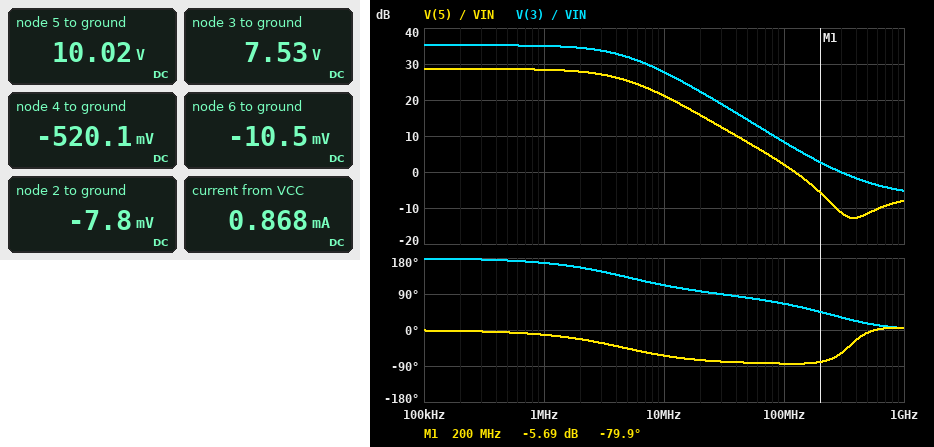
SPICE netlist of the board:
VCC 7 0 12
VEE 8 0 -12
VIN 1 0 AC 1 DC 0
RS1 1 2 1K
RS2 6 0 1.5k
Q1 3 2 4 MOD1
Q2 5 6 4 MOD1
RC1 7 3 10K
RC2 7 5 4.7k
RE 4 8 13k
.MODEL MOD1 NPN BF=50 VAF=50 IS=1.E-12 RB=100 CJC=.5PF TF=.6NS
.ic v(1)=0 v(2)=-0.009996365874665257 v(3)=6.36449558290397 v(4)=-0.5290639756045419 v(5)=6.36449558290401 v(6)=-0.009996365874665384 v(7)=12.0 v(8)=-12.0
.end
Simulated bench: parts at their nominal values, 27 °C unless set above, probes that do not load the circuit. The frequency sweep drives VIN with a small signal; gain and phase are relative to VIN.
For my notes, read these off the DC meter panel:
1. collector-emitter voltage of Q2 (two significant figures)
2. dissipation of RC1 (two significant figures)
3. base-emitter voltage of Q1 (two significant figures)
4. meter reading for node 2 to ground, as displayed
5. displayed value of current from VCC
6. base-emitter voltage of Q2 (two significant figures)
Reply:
11 V
2.0 mW
510 mV
-7.8 mV
0.868 mA
510 mV
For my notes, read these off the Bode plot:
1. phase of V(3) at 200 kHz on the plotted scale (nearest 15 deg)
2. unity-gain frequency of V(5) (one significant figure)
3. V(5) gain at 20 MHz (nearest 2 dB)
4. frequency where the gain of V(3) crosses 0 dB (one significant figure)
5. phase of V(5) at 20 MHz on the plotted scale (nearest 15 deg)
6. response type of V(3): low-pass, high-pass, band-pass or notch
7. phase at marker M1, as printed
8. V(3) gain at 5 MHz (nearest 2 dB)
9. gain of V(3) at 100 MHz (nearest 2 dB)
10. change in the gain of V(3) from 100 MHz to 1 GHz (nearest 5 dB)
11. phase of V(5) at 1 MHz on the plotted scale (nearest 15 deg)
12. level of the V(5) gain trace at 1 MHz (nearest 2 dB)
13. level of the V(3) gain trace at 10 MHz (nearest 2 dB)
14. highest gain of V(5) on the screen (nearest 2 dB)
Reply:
180 deg
100 MHz
16 dB
300 MHz
-75 deg
low-pass
-79.9 deg
32 dB
8 dB
-15 dB
-15 deg
28 dB
28 dB
28 dB
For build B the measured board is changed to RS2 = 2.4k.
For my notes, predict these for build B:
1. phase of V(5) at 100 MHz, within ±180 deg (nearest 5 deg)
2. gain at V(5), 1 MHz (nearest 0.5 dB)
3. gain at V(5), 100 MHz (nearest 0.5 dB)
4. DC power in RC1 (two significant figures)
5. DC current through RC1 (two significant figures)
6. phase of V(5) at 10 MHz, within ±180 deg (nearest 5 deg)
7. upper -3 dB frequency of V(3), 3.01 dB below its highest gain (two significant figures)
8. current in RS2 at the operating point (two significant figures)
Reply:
-80 deg
27.5 dB
-0.5 dB
2.3 mW
480 µA
-65 deg
4.1 MHz
6.4 µA
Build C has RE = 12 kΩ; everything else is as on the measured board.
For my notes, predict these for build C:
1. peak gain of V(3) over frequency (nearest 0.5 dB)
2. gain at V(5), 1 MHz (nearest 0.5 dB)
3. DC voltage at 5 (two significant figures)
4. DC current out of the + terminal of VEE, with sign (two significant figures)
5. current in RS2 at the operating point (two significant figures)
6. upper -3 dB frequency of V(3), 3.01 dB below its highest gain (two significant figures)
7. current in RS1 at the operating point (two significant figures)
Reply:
35.5 dB
29.0 dB
9.9 V
-960 µA
7.6 µA
4.4 MHz
8.5 µA
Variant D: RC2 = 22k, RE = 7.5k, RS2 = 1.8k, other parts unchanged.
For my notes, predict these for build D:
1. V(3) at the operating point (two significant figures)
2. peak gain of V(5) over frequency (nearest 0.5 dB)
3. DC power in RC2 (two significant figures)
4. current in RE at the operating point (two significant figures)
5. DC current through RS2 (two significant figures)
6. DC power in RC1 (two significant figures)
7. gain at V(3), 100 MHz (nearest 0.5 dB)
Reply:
2.7 V
11.0 dB
7.0 mW
1.5 mA
16 µA
8.6 mW
5.5 dB
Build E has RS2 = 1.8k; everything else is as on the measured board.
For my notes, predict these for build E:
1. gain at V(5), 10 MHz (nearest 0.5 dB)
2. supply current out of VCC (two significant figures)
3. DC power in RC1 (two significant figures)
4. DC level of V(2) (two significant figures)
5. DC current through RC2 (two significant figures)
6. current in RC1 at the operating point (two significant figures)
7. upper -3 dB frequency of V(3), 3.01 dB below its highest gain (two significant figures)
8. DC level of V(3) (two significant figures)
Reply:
20.5 dB
870 µA
2.1 mW
-8.0 mV
410 µA
460 µA
4.5 MHz
7.4 V
